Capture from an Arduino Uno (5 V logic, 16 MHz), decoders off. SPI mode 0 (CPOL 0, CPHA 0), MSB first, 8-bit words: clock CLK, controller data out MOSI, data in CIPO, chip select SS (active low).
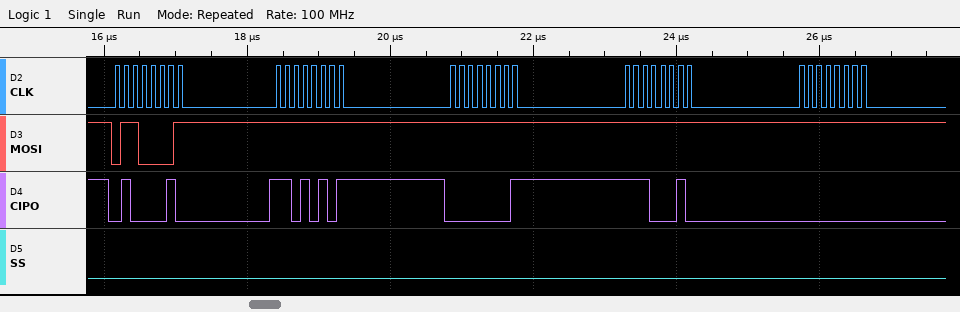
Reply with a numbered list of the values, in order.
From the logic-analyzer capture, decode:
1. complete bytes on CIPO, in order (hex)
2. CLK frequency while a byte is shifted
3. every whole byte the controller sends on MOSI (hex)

1. 42 D5 01 E2 00
2. 8 MHz
3. 61 FF FF FF FF
